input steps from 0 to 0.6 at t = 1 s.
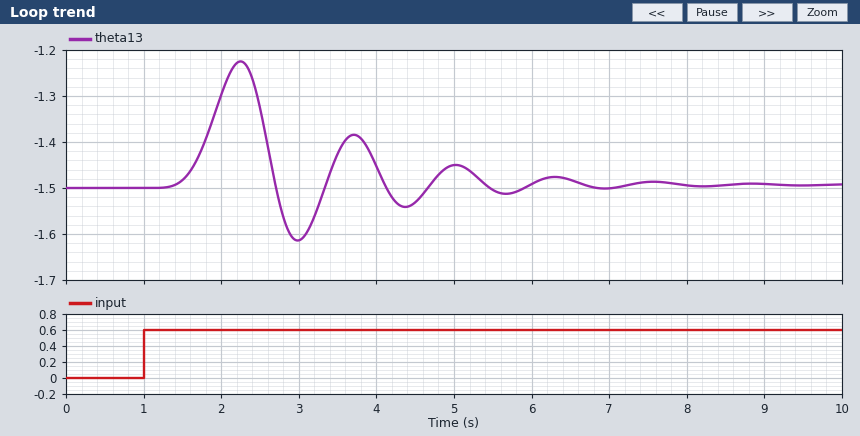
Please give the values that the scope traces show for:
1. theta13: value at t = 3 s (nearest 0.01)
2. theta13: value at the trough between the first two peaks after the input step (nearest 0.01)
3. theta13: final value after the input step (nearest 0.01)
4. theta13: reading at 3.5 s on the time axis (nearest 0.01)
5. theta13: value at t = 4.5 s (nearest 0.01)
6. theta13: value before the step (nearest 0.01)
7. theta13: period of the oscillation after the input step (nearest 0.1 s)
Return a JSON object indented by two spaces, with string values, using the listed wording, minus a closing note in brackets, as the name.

{
  "theta13: value at t = 3 s": "-1.61",
  "theta13: value at the trough between the first two peaks after the input step": "-1.61",
  "theta13: final value after the input step": "-1.49",
  "theta13: reading at 3.5 s on the time axis": "-1.43",
  "theta13: value at t = 4.5 s": "-1.53",
  "theta13: value before the step": "-1.50",
  "theta13: period of the oscillation after the input step": "1.5 s"
}
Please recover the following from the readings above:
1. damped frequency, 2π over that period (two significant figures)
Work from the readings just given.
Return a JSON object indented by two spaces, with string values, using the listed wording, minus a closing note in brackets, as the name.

{
  "damped frequency, 2π over that period": "4.2 rad/s"
}
